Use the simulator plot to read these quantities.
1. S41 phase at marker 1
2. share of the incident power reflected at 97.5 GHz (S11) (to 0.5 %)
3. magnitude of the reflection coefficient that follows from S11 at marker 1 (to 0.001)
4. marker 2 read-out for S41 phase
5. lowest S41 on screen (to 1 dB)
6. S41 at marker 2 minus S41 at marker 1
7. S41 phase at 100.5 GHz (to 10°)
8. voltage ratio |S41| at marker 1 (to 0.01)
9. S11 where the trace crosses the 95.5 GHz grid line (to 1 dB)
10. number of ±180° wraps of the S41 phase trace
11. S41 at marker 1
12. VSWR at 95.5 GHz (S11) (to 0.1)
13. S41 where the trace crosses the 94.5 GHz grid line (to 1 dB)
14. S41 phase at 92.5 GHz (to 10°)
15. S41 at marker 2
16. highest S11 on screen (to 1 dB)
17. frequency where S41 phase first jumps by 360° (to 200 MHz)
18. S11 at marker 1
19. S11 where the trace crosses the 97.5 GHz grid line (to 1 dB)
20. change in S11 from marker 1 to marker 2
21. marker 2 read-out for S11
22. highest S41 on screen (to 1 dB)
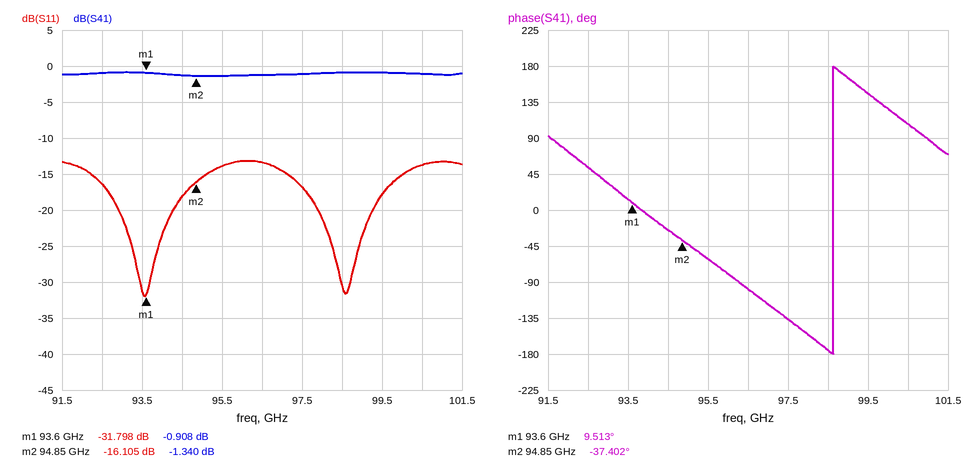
9.513°
2.0 %
0.026
-37.402°
-1 dB
-0.432 dB
110°
0.90
-14 dB
1
-0.908 dB
1.5
-1 dB
50°
-1.340 dB
-13 dB
98.6 GHz
-31.798 dB
-17 dB
15.693 dB
-16.105 dB
-1 dB
